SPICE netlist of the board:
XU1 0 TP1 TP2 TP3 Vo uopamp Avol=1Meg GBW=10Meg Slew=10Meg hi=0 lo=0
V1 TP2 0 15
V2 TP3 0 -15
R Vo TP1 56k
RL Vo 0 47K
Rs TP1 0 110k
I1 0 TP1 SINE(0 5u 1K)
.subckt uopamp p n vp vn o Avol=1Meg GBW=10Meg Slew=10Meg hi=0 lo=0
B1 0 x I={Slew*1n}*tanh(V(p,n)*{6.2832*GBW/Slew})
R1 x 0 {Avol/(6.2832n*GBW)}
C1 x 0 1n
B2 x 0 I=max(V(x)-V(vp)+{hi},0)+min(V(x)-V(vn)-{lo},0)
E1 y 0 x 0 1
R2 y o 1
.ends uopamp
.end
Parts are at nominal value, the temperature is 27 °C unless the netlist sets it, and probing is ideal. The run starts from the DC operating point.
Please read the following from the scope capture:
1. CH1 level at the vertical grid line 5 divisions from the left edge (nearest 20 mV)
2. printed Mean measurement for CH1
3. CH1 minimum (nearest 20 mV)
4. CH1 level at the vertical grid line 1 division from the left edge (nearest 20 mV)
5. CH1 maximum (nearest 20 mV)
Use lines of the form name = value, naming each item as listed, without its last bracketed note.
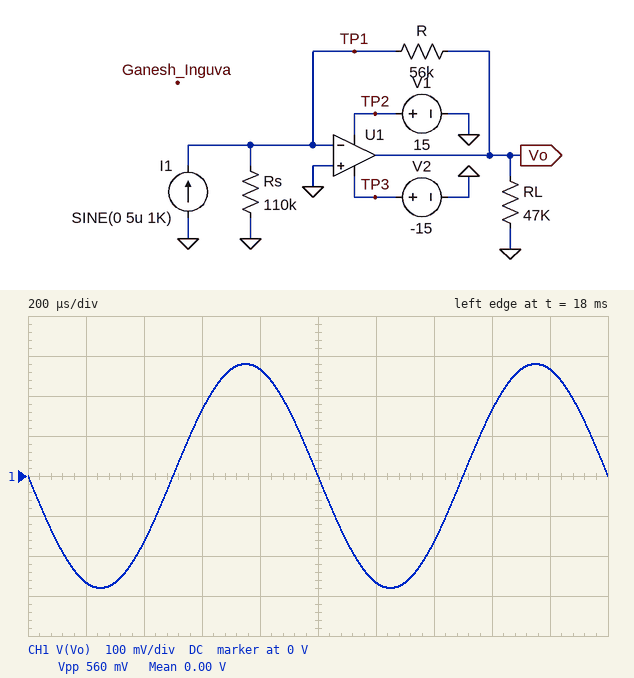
CH1 level at the vertical grid line 5 divisions from the left edge = 0 V
printed Mean measurement for CH1 = 0.00 V
CH1 minimum = -280 mV
CH1 level at the vertical grid line 1 division from the left edge = -260 mV
CH1 maximum = 280 mV
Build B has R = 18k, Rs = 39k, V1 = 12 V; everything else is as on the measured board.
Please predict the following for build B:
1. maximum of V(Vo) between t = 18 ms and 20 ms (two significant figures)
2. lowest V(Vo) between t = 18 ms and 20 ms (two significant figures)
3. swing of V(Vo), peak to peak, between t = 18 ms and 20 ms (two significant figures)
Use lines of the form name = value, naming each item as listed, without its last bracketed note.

maximum of V(Vo) between t = 18 ms and 20 ms = 90 mV
lowest V(Vo) between t = 18 ms and 20 ms = -90 mV
swing of V(Vo), peak to peak, between t = 18 ms and 20 ms = 180 mV
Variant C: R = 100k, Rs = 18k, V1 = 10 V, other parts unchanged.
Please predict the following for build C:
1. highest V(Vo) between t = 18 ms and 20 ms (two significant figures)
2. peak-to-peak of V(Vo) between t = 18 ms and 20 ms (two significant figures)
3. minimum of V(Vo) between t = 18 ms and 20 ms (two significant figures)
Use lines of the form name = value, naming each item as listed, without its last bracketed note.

highest V(Vo) between t = 18 ms and 20 ms = 500 mV
peak-to-peak of V(Vo) between t = 18 ms and 20 ms = 1.0 V
minimum of V(Vo) between t = 18 ms and 20 ms = -500 mV
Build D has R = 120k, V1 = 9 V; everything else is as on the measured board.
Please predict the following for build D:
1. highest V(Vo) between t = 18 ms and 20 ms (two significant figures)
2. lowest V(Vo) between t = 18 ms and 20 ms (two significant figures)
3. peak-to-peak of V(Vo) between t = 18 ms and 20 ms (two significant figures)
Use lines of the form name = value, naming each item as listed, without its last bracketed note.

highest V(Vo) between t = 18 ms and 20 ms = 600 mV
lowest V(Vo) between t = 18 ms and 20 ms = -600 mV
peak-to-peak of V(Vo) between t = 18 ms and 20 ms = 1.2 V
